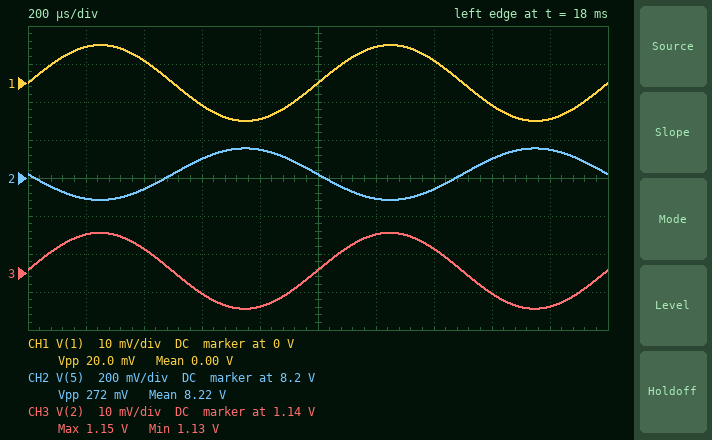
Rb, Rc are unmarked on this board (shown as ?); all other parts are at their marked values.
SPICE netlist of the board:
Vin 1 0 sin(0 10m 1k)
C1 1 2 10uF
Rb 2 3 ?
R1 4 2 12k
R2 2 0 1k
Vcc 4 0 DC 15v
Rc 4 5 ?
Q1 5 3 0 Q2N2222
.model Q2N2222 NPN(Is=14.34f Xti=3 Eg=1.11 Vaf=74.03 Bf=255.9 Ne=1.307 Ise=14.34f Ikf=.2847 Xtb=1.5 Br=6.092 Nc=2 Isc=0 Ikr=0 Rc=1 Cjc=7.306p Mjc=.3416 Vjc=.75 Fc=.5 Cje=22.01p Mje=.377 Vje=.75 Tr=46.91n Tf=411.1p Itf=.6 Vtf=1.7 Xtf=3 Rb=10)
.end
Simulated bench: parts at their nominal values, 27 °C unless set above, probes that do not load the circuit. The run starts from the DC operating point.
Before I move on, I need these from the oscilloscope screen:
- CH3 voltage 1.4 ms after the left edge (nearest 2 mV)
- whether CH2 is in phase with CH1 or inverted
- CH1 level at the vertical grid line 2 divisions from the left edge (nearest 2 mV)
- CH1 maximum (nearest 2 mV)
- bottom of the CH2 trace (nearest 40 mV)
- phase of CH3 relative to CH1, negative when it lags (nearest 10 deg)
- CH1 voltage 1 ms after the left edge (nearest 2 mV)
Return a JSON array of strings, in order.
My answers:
["1.146 V", "inverted", "6 mV", "10 mV", "8.08 V", "0 deg", "0 V"]
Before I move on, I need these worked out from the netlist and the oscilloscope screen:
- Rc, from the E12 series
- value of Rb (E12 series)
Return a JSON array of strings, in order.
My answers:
["2.7 kΩ", "33 kΩ"]
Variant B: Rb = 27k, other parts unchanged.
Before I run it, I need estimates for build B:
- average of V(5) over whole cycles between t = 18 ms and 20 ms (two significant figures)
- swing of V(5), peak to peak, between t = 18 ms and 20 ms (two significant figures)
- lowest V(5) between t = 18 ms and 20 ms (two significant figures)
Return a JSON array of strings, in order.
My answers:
["6.9 V", "320 mV", "6.7 V"]
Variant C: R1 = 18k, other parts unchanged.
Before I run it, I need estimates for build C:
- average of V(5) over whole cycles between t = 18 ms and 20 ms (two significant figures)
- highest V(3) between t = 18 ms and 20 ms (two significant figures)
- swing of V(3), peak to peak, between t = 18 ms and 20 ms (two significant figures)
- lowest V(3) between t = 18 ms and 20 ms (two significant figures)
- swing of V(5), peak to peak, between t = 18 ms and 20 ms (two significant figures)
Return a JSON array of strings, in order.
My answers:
["13 V", "640 mV", "3.2 mV", "630 mV", "250 mV"]
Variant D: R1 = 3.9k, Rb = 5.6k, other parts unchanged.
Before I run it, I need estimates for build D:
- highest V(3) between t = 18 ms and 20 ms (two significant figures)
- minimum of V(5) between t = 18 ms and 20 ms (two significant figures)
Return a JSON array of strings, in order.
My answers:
["700 mV", "42 mV"]
